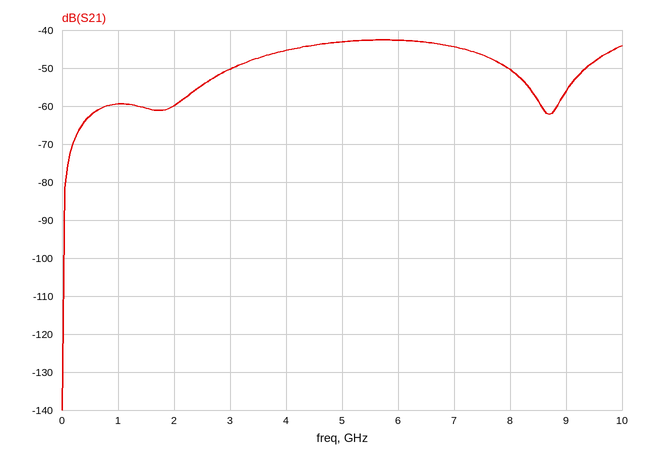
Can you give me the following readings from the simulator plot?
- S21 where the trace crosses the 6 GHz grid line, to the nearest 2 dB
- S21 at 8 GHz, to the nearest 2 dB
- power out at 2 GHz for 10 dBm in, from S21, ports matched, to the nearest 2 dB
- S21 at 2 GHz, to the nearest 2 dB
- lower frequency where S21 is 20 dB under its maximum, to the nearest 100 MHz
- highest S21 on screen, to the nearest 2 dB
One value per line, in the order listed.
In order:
-42 dB
-50 dB
-50 dBm
-60 dB
500 MHz
-42 dB
